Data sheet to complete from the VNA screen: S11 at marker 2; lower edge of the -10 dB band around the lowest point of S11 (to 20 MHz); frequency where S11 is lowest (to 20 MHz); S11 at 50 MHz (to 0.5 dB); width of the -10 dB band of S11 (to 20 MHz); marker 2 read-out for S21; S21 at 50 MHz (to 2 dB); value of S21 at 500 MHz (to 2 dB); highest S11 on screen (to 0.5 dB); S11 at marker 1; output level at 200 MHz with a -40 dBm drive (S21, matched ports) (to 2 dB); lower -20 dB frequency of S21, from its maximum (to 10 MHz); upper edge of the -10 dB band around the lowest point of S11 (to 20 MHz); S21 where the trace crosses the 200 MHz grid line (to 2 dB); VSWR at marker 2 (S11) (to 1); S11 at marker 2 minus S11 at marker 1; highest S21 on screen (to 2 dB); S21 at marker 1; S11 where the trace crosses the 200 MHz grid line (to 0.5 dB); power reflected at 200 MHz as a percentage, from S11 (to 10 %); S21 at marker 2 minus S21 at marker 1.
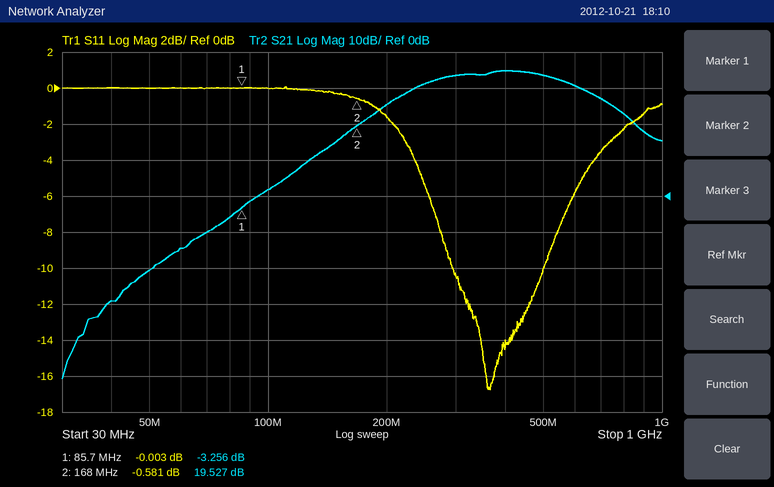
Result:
-0.581 dB
300 MHz
360 MHz
0.0 dB
200 MHz
19.527 dB
-20 dB
34 dB
0.0 dB
-0.003 dB
-14 dBm
150 MHz
500 MHz
26 dB
30
-0.578 dB
34 dB
-3.256 dB
-1.5 dB
70 %
22.783 dB
